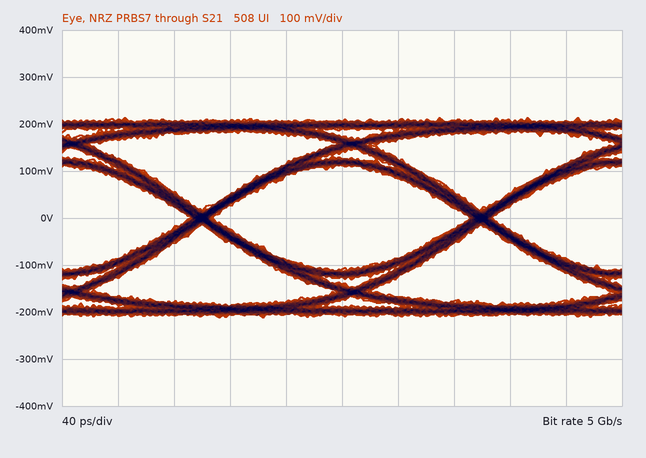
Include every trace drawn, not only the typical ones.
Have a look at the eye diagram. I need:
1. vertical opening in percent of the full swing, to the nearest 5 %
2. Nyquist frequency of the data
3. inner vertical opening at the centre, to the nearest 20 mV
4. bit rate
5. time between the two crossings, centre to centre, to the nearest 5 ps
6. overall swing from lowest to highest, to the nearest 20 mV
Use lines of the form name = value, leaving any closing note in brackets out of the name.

vertical opening in percent of the full swing, to the nearest 5 % = 50 %
Nyquist frequency of the data = 2.5 GHz
inner vertical opening at the centre, to the nearest 20 mV = 220 mV
bit rate = 5 Gb/s
time between the two crossings, centre to centre, to the nearest 5 ps = 200 ps
overall swing from lowest to highest, to the nearest 20 mV = 420 mV
